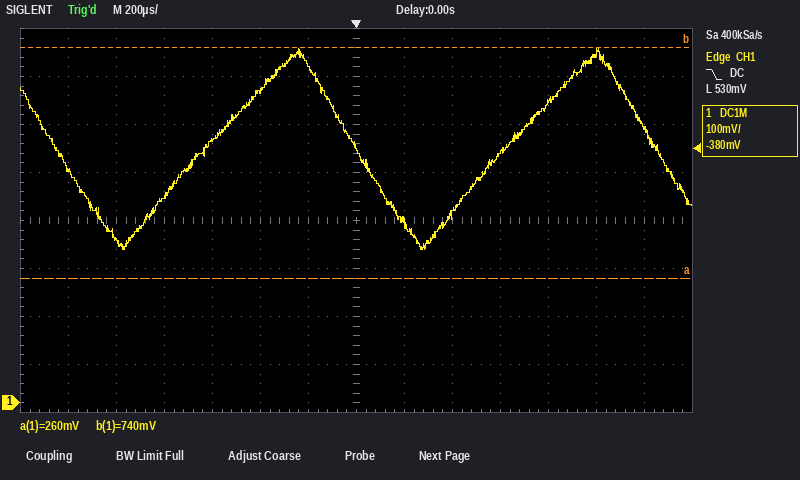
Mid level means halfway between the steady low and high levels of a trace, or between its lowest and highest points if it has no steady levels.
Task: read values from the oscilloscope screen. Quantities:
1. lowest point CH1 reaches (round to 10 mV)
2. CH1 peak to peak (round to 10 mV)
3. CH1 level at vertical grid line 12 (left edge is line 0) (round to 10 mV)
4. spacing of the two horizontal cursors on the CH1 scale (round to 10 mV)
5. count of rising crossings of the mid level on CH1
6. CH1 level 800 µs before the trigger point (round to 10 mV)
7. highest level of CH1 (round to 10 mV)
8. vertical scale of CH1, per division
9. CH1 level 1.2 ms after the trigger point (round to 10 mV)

320 mV
420 mV
730 mV
480 mV
2
430 mV
740 mV
100 mV
570 mV
